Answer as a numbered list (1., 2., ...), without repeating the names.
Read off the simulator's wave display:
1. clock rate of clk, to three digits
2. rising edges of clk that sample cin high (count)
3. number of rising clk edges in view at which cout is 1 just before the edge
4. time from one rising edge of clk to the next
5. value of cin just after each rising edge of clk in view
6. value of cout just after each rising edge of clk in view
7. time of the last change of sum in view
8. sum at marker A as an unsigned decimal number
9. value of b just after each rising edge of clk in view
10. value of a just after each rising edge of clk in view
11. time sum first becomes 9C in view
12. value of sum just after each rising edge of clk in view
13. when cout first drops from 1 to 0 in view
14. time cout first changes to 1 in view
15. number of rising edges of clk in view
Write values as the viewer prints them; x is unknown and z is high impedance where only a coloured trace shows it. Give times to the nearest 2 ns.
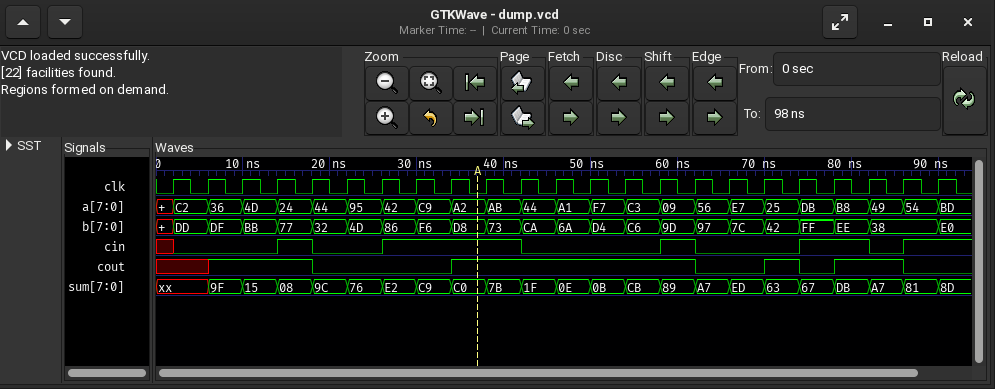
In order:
1. 250 MHz
2. 9
3. 13
4. 4 ns
5. 0 0 0 1 0 0 1 1 1 1 0 0 0 0 1 0 0 0 1 1 0 1 1
6. x 1 1 1 0 0 0 0 1 1 1 1 1 1 1 0 0 1 0 1 1 0 0
7. 90 ns
8. 192
9. DD, DF, BB, 77, 32, 4D, 86, F6, D8, 73, CA, 6A, D4, C6, 9D, 97, 7C, 42, FF, EE, 38, 38, E0
10. C2, 36, 4D, 24, 44, 95, 42, C9, A2, AB, 44, A1, F7, C3, 09, 56, E7, 25, DB, B8, 49, 54, BD
11. 18 ns
12. xx, 9F, 15, 08, 9C, 76, E2, C9, C0, 7B, 1F, 0E, 0B, CB, 89, A7, ED, 63, 67, DB, A7, 81, 8D
13. 18 ns
14. 6 ns
15. 23
